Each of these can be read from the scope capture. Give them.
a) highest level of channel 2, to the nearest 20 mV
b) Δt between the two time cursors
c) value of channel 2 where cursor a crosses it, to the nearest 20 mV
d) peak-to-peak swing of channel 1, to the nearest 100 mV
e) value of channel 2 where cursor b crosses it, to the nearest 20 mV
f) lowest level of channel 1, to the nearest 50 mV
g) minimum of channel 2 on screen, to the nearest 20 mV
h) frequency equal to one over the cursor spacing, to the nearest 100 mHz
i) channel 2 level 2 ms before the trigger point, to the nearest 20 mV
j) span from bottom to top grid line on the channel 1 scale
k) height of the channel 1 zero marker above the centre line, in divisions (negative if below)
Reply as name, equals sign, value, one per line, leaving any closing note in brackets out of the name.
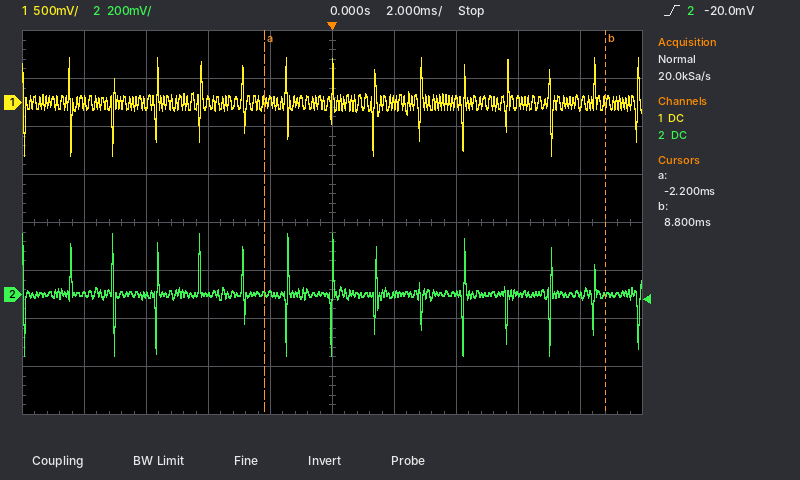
highest level of channel 2, to the nearest 20 mV = 260 mV
Δt between the two time cursors = 11.0 ms
value of channel 2 where cursor a crosses it, to the nearest 20 mV = 0 mV
peak-to-peak swing of channel 1, to the nearest 100 mV = 1.00 V
value of channel 2 where cursor b crosses it, to the nearest 20 mV = 0 mV
lowest level of channel 1, to the nearest 50 mV = -550 mV
minimum of channel 2 on screen, to the nearest 20 mV = -260 mV
frequency equal to one over the cursor spacing, to the nearest 100 mHz = 90.9 Hz
channel 2 level 2 ms before the trigger point, to the nearest 20 mV = 0 mV
span from bottom to top grid line on the channel 1 scale = 4 V
height of the channel 1 zero marker above the centre line, in divisions = +2.5 div
